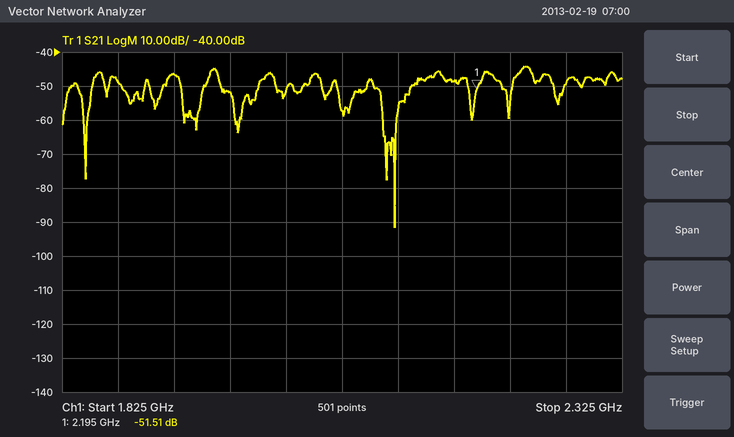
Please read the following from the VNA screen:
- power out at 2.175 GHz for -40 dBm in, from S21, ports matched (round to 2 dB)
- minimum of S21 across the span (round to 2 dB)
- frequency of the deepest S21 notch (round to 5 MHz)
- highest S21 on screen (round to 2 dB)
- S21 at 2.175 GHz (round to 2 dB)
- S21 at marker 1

-88 dBm
-92 dB
2.120 GHz
-44 dB
-48 dB
-51.51 dB
